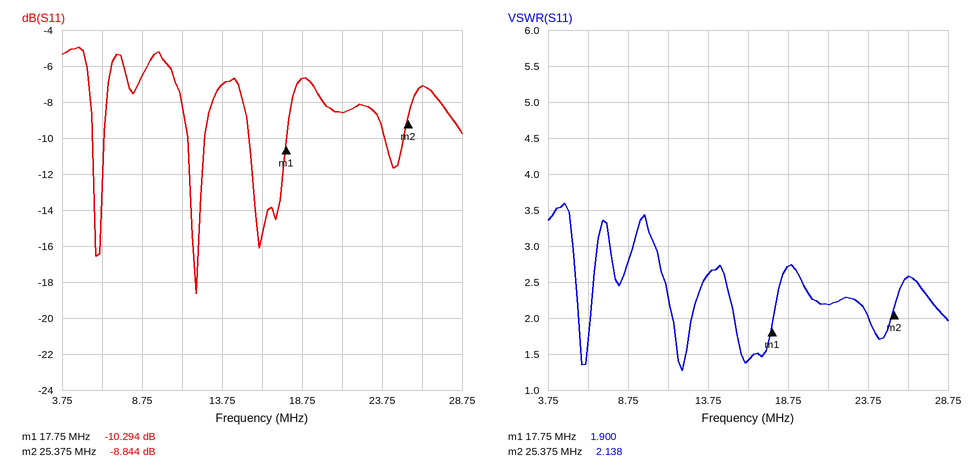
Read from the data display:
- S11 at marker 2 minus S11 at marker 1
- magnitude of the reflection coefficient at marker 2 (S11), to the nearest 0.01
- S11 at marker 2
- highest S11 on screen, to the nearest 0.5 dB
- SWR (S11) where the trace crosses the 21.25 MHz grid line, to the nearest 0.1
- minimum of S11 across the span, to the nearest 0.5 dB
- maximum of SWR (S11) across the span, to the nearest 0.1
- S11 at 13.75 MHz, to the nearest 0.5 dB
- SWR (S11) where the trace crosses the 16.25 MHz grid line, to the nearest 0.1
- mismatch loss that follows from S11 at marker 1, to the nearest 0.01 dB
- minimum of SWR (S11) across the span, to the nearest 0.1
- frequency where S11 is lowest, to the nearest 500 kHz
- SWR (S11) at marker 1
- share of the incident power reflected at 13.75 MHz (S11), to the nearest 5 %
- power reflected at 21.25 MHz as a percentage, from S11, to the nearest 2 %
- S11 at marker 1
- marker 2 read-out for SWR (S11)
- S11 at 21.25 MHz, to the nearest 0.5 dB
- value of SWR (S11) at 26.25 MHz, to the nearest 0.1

1.450 dB
0.36
-8.844 dB
-5.0 dB
2.2
-18.5 dB
3.6
-7.0 dB
1.4
0.43 dB
1.3
12.0 MHz
1.900
20 %
14 %
-10.294 dB
2.138
-8.5 dB
2.6
